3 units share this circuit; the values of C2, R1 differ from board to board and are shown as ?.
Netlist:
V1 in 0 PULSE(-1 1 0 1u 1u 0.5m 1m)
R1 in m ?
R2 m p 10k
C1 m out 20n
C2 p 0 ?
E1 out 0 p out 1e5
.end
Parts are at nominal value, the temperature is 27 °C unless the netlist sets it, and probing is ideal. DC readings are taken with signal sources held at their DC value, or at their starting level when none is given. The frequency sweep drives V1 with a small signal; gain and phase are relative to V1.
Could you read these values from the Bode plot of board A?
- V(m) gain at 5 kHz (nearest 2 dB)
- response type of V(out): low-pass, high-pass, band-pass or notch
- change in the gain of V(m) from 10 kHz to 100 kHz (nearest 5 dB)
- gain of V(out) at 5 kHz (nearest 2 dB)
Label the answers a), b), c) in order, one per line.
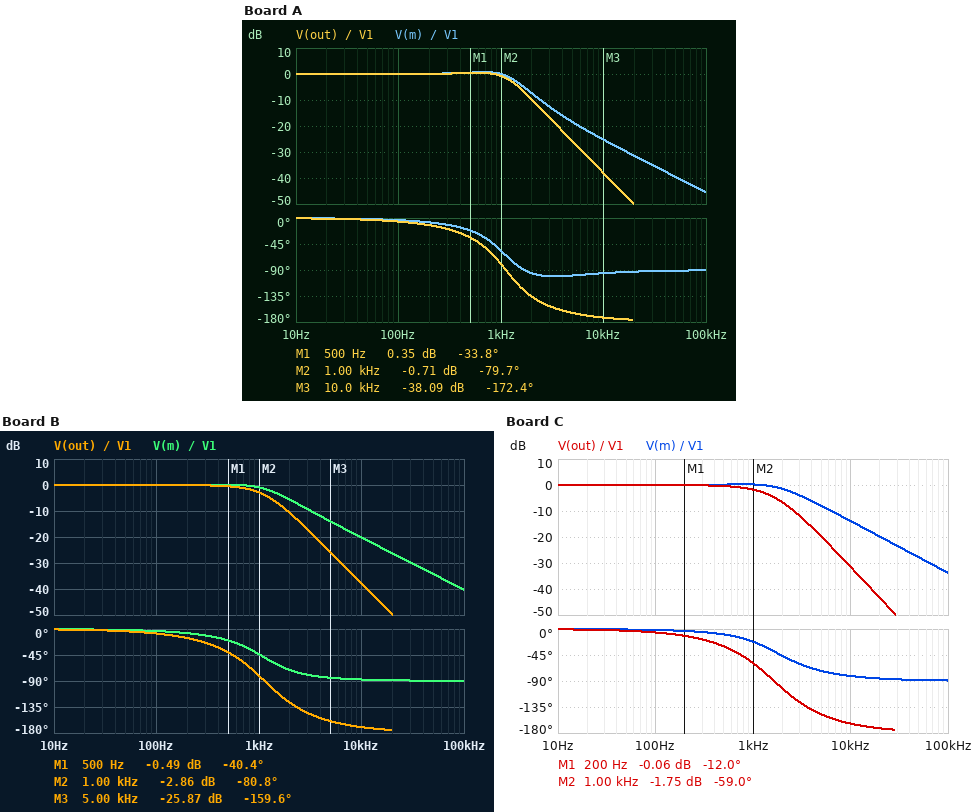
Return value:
a) -18 dB
b) low-pass
c) -20 dB
d) -26 dB
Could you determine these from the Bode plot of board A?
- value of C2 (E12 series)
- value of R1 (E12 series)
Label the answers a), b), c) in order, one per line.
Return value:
a) 6.8 nF
b) 15 kΩ
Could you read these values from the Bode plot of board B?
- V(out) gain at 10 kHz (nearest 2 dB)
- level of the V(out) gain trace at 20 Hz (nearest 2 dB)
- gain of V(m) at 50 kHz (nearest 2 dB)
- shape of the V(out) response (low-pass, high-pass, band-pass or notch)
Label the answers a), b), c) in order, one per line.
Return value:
a) -38 dB
b) 0 dB
c) -34 dB
d) low-pass
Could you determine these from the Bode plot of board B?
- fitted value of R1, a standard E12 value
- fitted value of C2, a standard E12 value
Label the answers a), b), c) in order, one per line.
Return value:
a) 8.2 kΩ
b) 12 nF
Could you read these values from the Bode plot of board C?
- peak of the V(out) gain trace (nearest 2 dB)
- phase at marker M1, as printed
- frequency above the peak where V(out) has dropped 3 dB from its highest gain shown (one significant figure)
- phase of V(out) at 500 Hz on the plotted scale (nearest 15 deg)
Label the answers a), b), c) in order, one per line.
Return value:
a) 0 dB
b) -12.0 deg
c) 1 kHz
d) -30 deg
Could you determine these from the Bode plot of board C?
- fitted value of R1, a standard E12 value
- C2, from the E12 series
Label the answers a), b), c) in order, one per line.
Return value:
a) 3.9 kΩ
b) 12 nF
